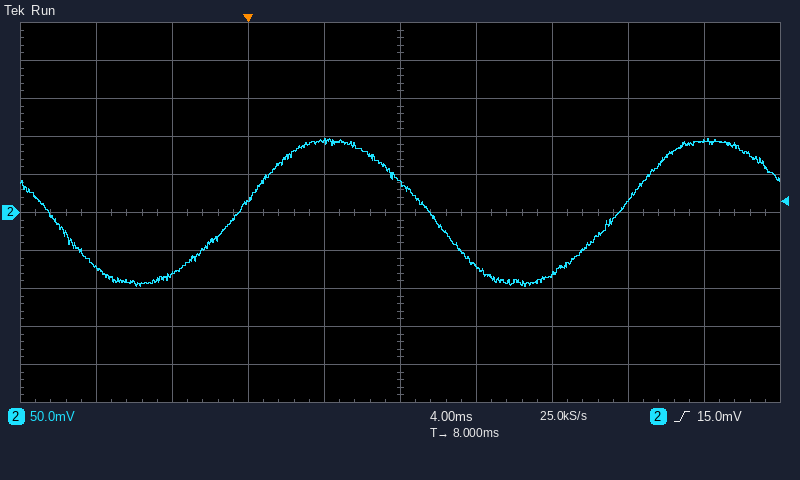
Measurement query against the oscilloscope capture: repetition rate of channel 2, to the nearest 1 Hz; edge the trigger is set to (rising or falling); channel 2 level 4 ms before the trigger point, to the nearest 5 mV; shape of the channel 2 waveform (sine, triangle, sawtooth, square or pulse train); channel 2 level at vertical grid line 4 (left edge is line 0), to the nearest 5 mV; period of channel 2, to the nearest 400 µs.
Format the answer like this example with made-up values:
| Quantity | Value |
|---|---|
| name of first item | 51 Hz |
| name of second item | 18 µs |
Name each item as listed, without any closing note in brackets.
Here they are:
| Quantity | Value |
|---|---|
| repetition rate of channel 2, to the nearest 1 Hz | 50 Hz |
| edge the trigger is set to | rising |
| channel 2 level 4 ms before the trigger point, to the nearest 5 mV | -80 mV |
| shape of the channel 2 waveform | sine |
| channel 2 level at vertical grid line 4 (left edge is line 0), to the nearest 5 mV | 95 mV |
| period of channel 2, to the nearest 400 µs | 20.0 ms |
